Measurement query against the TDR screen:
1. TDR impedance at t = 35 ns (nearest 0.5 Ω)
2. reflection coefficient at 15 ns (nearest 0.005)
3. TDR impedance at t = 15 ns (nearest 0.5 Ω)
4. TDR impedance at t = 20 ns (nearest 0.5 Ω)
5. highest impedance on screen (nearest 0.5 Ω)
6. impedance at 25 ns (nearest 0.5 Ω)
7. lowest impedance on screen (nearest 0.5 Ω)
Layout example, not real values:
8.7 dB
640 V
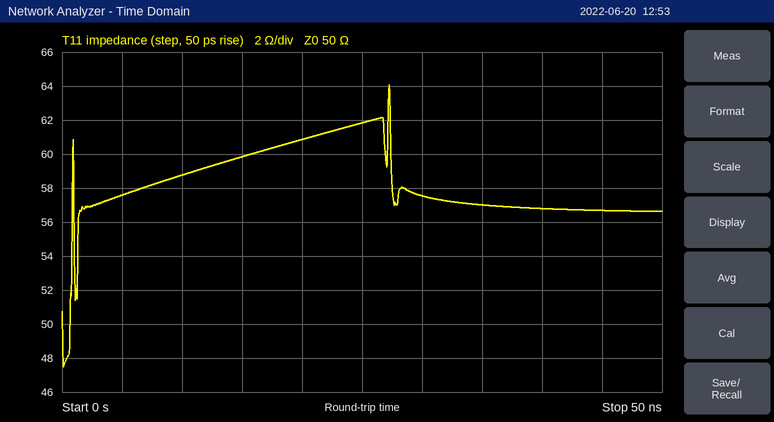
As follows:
57.0 Ω
+0.090
60.0 Ω
61.0 Ω
64.0 Ω
62.0 Ω
47.5 Ω
